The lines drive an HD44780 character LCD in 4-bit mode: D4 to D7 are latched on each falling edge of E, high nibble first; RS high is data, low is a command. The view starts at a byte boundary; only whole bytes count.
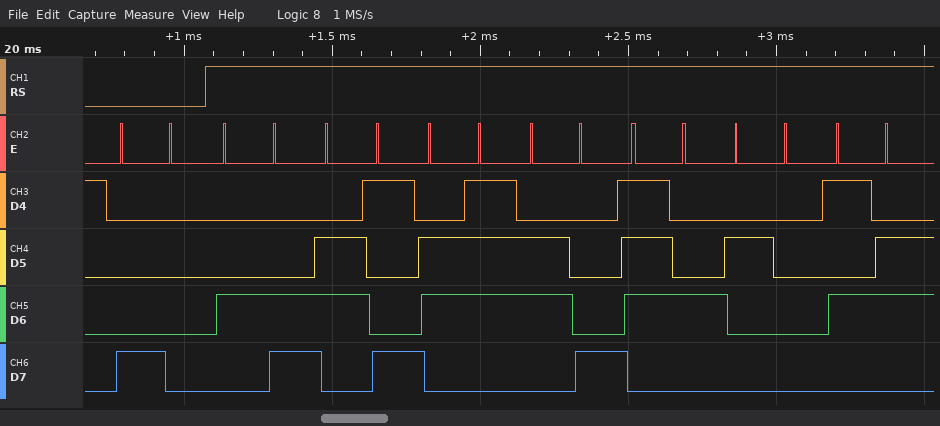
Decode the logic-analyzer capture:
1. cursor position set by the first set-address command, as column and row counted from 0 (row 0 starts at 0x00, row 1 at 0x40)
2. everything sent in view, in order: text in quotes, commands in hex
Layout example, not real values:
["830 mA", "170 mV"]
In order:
["column 0, row 0", "0x80 \"Light V\""]
